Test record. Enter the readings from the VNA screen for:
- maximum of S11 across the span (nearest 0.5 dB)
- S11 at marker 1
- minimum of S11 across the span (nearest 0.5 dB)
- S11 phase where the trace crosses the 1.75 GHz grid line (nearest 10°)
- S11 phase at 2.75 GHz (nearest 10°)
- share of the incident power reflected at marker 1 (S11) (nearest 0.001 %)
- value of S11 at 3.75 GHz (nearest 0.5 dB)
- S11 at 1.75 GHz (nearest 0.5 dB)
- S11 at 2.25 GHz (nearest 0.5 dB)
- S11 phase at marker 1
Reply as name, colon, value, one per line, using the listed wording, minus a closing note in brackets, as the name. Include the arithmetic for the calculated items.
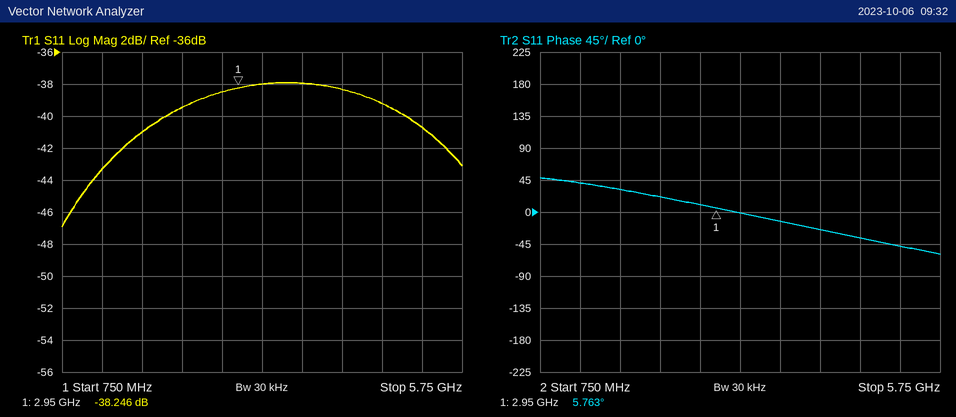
maximum of S11 across the span: -38.0 dB
S11 at marker 1: -38.246 dB
minimum of S11 across the span: -47.0 dB
S11 phase where the trace crosses the 1.75 GHz grid line: 30°
S11 phase at 2.75 GHz: 10°
share of the incident power reflected at marker 1 (S11): 10^(-38.246/10) ≈ 0.015 %
value of S11 at 3.75 GHz: -38.0 dB
S11 at 1.75 GHz: -41.0 dB
S11 at 2.25 GHz: -39.5 dB
S11 phase at marker 1: 5.763°
